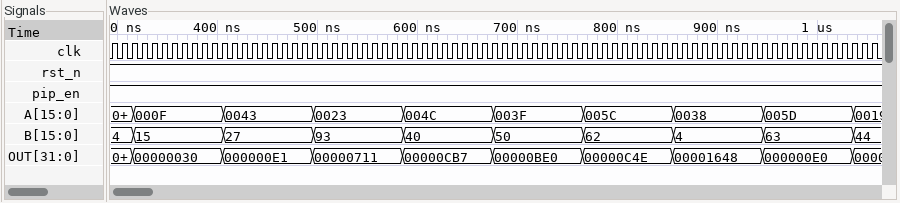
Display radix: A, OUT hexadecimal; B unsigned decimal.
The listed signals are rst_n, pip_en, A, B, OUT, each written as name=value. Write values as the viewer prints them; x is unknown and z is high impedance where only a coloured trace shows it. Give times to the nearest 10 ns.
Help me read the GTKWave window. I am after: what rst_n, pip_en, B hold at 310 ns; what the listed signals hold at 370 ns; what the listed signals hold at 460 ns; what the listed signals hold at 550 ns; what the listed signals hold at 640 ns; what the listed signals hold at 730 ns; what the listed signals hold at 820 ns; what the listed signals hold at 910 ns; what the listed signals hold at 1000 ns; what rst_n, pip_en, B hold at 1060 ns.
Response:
rst_n=1, pip_en=1, B=4
rst_n=1, pip_en=1, A=000F, B=15, OUT=00000030
rst_n=1, pip_en=1, A=0043, B=27, OUT=000000E1
rst_n=1, pip_en=1, A=0023, B=93, OUT=00000711
rst_n=1, pip_en=1, A=004C, B=40, OUT=00000CB7
rst_n=1, pip_en=1, A=003F, B=50, OUT=00000BE0
rst_n=1, pip_en=1, A=005C, B=62, OUT=00000C4E
rst_n=1, pip_en=1, A=0038, B=4, OUT=00001648
rst_n=1, pip_en=1, A=005D, B=63, OUT=000000E0
rst_n=1, pip_en=1, B=44
